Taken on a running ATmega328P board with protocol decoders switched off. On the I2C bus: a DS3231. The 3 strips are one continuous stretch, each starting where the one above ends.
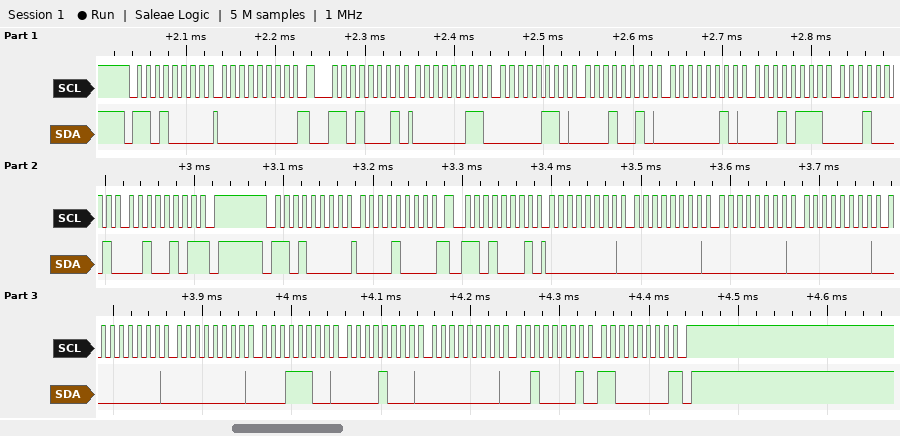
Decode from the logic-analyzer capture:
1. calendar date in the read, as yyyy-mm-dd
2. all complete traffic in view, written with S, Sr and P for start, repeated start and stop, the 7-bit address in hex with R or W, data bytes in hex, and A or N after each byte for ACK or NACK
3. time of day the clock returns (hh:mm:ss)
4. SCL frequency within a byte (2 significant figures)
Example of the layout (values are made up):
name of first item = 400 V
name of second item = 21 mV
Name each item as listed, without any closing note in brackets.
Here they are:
calendar date in the read, as yyyy-mm-dd = 2025-11-17
all complete traffic in view, written with S, Sr and P for start, repeated start and stop, the 7-bit address in hex with R or W, data bytes in hex, and A or N after each byte for ACK or NACK = S 68W A 00 A Sr 68R A 03 A 06 A 12 A 02 A 17 A 11 A 25 N P S 68W A 08 A Sr 68R A 00 A 00 A 00 A 00 A 00 A 00 A 1C A 08 A 00 A 21 A C0 N P
time of day the clock returns = 12:06:03
SCL frequency within a byte = 100 kHz
